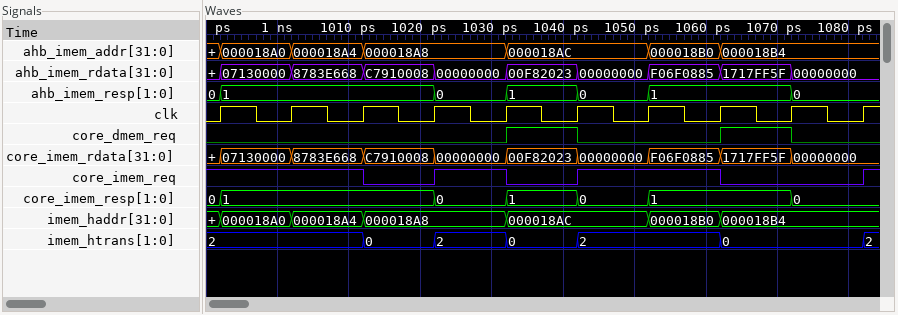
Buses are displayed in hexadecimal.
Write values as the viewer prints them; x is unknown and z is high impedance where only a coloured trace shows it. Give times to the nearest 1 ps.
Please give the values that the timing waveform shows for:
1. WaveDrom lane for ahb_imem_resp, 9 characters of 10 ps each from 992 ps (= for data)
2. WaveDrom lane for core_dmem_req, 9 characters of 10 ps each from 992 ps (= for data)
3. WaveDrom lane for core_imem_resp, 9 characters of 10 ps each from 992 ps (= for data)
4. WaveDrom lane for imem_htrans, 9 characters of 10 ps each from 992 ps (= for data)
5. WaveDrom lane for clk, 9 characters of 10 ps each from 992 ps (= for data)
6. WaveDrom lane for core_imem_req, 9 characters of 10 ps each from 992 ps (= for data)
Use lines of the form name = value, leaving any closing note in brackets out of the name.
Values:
WaveDrom lane for ahb_imem_resp, 9 characters of 10 ps each from 992 ps = {name: 'ahb_imem_resp', wave: '=..====.=', data: '1 0 1 0 1 0'}
WaveDrom lane for core_dmem_req, 9 characters of 10 ps each from 992 ps = {name: 'core_dmem_req', wave: '0...10.10'}
WaveDrom lane for core_imem_resp, 9 characters of 10 ps each from 992 ps = {name: 'core_imem_resp', wave: '=..====.=', data: '1 0 1 0 1 0'}
WaveDrom lane for imem_htrans, 9 characters of 10 ps each from 992 ps = {name: 'imem_htrans', wave: '=.====.=.', data: '2 0 2 0 2 0'}
WaveDrom lane for clk, 9 characters of 10 ps each from 992 ps = {name: 'clk', wave: 'p........'}
WaveDrom lane for core_imem_req, 9 characters of 10 ps each from 992 ps = {name: 'core_imem_req', wave: '1.0101.0.'}
